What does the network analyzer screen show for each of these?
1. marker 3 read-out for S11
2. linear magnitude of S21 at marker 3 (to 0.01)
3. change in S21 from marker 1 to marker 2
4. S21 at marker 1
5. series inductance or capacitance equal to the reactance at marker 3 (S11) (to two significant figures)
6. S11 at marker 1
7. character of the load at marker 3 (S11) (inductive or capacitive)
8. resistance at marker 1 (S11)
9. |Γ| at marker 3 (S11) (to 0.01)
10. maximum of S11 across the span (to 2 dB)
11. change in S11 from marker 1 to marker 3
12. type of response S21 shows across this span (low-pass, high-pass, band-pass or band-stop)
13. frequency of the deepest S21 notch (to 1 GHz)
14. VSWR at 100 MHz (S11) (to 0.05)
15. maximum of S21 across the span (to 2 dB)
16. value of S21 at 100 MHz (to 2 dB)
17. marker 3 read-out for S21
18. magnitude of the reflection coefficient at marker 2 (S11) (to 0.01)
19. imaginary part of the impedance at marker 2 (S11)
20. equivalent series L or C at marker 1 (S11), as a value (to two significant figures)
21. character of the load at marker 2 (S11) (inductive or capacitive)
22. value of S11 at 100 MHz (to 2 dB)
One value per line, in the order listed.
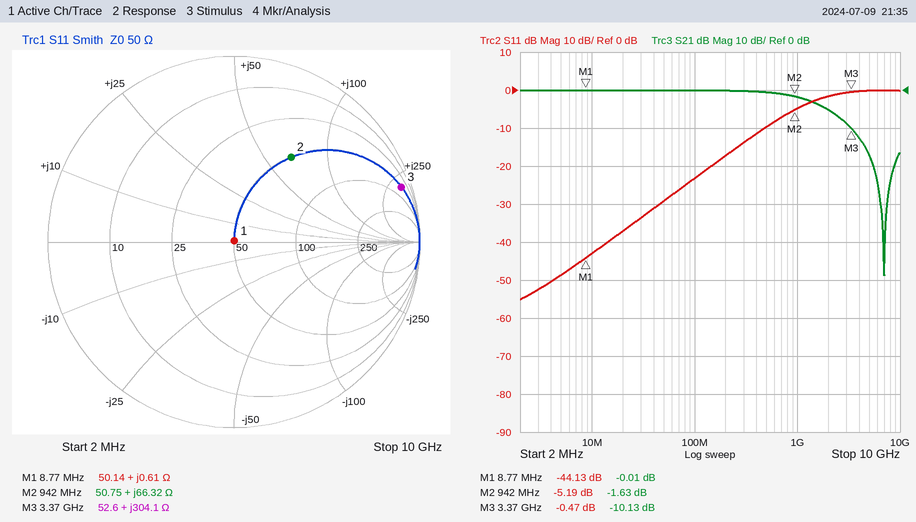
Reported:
-0.47 dB
0.31
-1.62 dB
-0.01 dB
14 nH
-44.13 dB
inductive
50.14 Ω
0.95
0 dB
43.66 dB
low-pass
7 GHz
1.15
0 dB
0 dB
-10.13 dB
0.55
+66.32 Ω
11 nH
inductive
-24 dB
